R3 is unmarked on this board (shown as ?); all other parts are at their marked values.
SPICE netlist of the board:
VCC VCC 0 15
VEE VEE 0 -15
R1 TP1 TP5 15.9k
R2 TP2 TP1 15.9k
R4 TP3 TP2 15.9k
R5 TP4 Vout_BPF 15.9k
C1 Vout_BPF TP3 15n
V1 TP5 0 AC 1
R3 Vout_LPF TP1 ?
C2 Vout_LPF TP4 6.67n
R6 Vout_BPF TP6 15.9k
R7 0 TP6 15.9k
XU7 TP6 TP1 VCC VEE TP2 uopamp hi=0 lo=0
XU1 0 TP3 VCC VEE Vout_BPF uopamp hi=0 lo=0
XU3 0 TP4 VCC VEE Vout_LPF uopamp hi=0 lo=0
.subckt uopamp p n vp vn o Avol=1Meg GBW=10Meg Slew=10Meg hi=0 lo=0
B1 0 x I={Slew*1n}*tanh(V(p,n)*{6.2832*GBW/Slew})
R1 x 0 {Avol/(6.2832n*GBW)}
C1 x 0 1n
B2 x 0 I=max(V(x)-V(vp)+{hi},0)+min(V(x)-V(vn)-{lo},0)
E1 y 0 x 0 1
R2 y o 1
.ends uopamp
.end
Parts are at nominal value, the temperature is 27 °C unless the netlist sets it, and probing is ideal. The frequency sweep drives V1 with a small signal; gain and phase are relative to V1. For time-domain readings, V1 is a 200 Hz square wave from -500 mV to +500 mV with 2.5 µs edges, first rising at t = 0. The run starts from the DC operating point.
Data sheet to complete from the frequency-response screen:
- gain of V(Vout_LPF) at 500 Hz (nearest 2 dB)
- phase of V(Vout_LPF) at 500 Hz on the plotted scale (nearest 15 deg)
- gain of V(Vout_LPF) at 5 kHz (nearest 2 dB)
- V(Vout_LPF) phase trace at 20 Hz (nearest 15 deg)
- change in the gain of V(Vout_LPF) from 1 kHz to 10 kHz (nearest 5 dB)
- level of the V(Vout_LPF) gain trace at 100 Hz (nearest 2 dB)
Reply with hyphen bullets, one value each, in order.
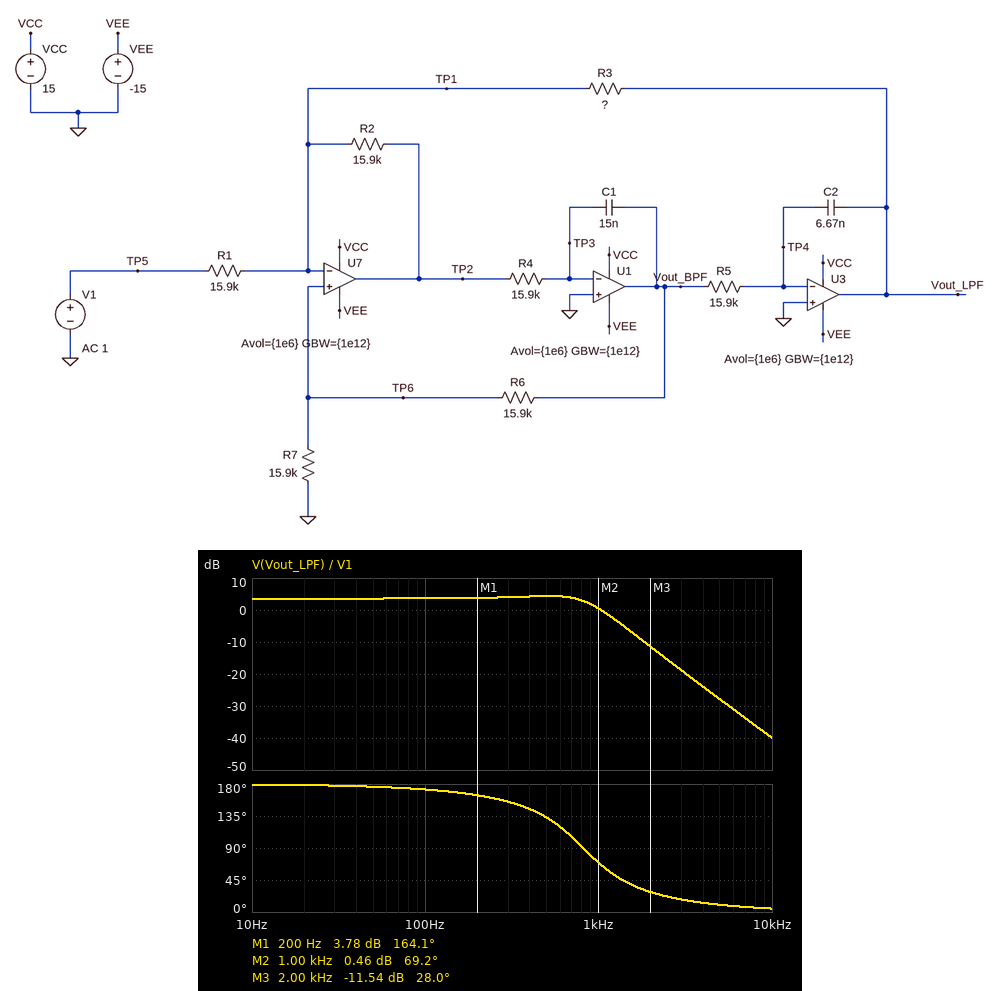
- 4 dB
- 135 deg
- -28 dB
- 180 deg
- -40 dB
- 4 dB
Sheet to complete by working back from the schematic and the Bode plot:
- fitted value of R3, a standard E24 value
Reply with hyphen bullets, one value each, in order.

- 24 kΩ
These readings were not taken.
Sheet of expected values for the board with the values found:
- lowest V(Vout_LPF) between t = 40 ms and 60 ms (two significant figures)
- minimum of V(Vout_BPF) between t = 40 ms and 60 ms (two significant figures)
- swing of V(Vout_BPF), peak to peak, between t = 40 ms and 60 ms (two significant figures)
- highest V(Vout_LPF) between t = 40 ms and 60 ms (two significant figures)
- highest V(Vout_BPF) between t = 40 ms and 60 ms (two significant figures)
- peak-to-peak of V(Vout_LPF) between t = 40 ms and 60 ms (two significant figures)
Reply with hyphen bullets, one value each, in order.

- -950 mV
- -430 mV
- 860 mV
- 950 mV
- 430 mV
- 1.9 V
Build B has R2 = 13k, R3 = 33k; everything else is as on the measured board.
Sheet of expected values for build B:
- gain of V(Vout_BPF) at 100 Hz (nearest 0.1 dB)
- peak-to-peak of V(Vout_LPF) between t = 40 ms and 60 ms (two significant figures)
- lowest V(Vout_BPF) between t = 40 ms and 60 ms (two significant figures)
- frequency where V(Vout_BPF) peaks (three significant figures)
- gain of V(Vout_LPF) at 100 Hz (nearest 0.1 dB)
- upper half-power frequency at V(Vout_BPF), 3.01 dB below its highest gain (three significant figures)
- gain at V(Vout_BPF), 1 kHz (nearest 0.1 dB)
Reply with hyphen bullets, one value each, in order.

- -17.1 dB
- 2.5 V
- -440 mV
- 628 Hz
- 6.4 dB
- 1.10 kHz
- -4.9 dB
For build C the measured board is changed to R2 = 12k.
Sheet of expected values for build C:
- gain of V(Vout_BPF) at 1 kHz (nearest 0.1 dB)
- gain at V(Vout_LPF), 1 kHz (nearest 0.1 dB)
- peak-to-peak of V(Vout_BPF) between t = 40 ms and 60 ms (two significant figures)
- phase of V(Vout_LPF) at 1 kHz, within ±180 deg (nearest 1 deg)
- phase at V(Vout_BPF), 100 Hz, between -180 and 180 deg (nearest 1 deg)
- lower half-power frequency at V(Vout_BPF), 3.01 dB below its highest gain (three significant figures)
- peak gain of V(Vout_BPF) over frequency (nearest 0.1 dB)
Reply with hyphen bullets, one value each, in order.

- -5.1 dB
- -1.5 dB
- 760 mV
- 56 deg
- 81 deg
- 425 Hz
- -3.5 dB
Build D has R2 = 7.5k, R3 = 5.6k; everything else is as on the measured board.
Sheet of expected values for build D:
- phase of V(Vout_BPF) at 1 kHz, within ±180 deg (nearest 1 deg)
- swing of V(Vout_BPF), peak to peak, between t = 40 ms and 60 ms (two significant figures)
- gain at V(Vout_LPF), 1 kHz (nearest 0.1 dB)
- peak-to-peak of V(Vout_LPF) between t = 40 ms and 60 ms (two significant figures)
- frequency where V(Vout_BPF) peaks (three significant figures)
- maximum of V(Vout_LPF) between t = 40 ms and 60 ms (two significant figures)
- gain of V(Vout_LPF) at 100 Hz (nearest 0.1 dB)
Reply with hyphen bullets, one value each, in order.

- 20 deg
- 330 mV
- -6.5 dB
- 530 mV
- 1.16 kHz
- 260 mV
- -9.0 dB
